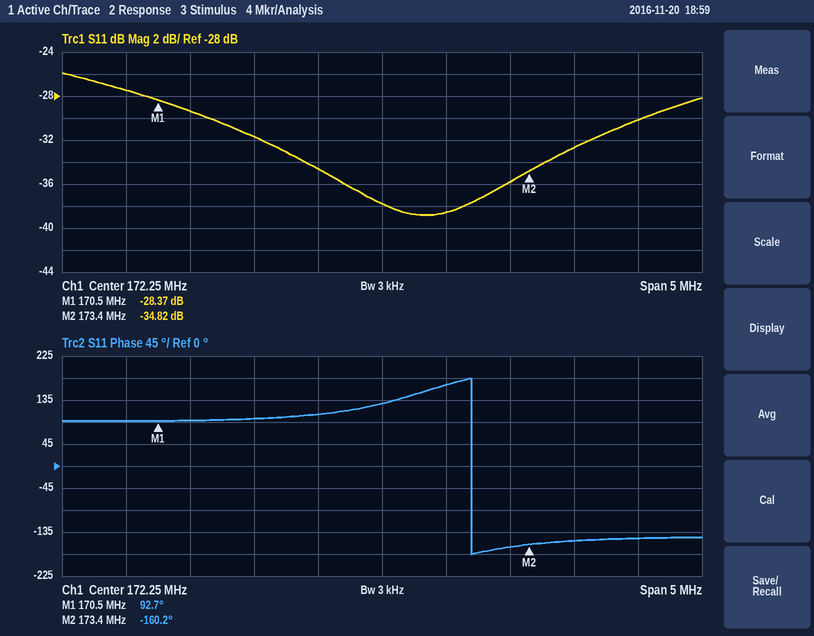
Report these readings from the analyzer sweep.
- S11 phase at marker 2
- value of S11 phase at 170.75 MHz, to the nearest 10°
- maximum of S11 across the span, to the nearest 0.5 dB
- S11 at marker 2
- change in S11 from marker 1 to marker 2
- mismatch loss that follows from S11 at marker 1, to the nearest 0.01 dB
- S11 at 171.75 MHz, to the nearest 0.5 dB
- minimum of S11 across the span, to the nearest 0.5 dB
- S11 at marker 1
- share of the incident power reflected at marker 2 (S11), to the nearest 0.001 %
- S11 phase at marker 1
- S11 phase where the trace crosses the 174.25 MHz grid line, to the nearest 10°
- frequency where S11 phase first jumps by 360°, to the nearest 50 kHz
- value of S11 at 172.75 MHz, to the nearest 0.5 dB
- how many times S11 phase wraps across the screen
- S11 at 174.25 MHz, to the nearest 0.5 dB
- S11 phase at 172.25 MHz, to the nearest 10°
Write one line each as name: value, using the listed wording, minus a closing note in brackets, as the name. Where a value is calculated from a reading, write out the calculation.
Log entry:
S11 phase at marker 2: -160.2°
value of S11 phase at 170.75 MHz, to the nearest 10°: 90°
maximum of S11 across the span, to the nearest 0.5 dB: -26.0 dB
S11 at marker 2: -34.82 dB
change in S11 from marker 1 to marker 2: -34.82 − (-28.37) = -6.45 dB
mismatch loss that follows from S11 at marker 1, to the nearest 0.01 dB: −10 log10(1 − 10^(-28.37/10)) ≈ 0.01 dB
S11 at 171.75 MHz, to the nearest 0.5 dB: -34.5 dB
minimum of S11 across the span, to the nearest 0.5 dB: -39.0 dB
S11 at marker 1: -28.37 dB
share of the incident power reflected at marker 2 (S11), to the nearest 0.001 %: 10^(-34.82/10) ≈ 0.033 %
S11 phase at marker 1: 92.7°
S11 phase where the trace crosses the 174.25 MHz grid line, to the nearest 10°: -150°
frequency where S11 phase first jumps by 360°, to the nearest 50 kHz: 172.95 MHz
value of S11 at 172.75 MHz, to the nearest 0.5 dB: -38.5 dB
how many times S11 phase wraps across the screen: 1
S11 at 174.25 MHz, to the nearest 0.5 dB: -30.0 dB
S11 phase at 172.25 MHz, to the nearest 10°: 130°
